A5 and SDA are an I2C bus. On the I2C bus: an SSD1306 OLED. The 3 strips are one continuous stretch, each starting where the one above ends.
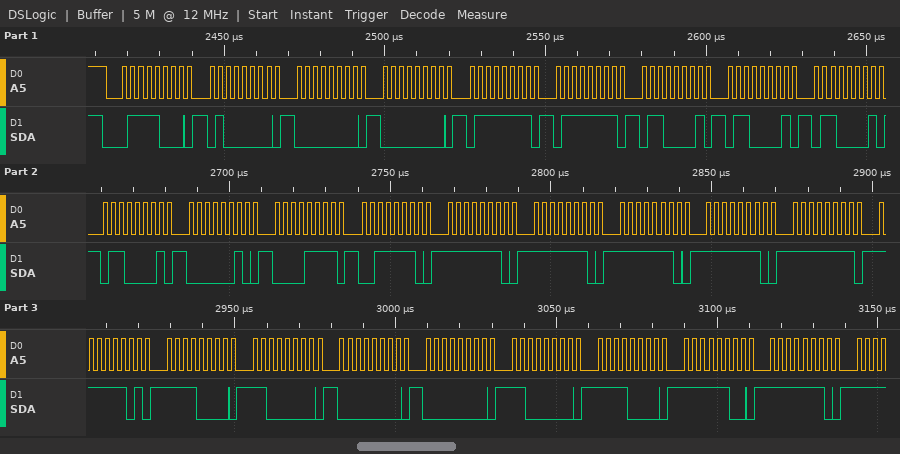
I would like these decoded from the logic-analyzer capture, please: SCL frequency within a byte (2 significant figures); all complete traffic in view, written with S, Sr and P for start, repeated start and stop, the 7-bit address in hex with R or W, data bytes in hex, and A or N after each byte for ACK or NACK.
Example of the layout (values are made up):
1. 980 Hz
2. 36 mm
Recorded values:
1. 400 kHz
2. S 3CW A 40 A 00 A 00 A 7F A 7F A 61 A 61 A 61 A 61 A 02 A 0F A 3E A FE A FE A FE A FE A FF A FD A F0 A C0 A 00 A 00 A C0 A F0 A FC A FE A
